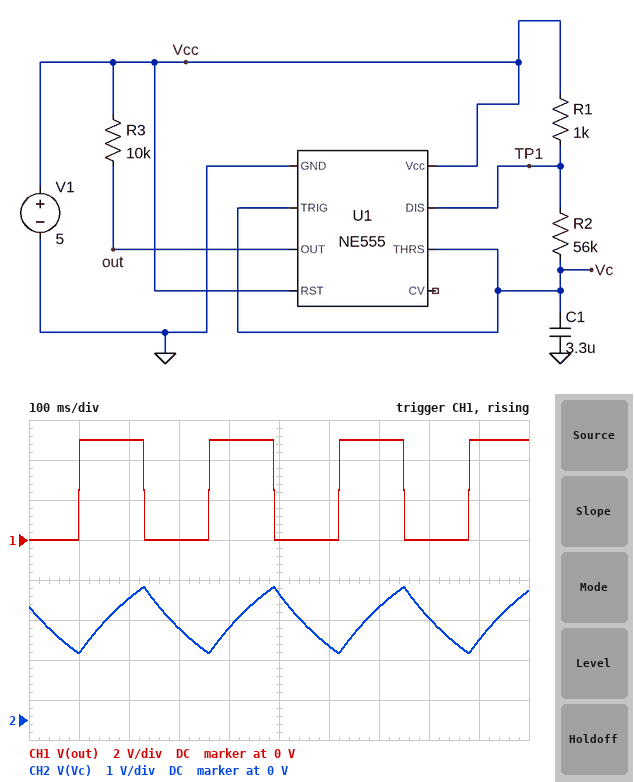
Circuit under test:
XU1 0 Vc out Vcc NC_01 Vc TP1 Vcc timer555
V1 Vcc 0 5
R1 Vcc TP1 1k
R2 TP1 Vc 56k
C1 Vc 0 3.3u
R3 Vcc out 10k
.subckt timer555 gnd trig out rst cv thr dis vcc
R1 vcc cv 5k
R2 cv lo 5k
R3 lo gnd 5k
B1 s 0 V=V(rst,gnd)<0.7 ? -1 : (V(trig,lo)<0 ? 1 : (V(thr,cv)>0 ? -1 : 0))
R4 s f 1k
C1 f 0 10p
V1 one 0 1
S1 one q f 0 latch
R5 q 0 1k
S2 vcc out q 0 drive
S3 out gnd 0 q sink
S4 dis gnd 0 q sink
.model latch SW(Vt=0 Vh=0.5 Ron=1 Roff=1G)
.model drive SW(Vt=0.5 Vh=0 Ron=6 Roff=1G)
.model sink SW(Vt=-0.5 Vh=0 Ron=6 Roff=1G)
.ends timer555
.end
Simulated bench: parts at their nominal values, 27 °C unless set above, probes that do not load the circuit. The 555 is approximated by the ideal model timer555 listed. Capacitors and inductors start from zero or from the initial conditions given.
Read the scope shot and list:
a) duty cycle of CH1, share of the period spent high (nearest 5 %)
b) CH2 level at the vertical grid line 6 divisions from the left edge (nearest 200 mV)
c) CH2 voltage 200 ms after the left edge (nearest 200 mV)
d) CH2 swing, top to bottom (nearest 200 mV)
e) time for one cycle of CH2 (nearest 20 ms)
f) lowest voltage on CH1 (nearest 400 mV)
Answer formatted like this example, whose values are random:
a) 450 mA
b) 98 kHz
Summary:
a) 50 %
b) 1.8 V
c) 3.0 V
d) 1.6 V
e) 260 ms
f) 0 V
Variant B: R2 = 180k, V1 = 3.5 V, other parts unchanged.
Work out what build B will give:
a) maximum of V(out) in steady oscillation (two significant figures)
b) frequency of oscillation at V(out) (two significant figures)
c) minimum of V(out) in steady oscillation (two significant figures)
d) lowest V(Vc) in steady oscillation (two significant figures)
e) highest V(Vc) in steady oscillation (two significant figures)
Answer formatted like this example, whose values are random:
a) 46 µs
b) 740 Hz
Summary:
a) 3.5 V
b) 1.2 Hz
c) 2.1 mV
d) 1.2 V
e) 2.3 V
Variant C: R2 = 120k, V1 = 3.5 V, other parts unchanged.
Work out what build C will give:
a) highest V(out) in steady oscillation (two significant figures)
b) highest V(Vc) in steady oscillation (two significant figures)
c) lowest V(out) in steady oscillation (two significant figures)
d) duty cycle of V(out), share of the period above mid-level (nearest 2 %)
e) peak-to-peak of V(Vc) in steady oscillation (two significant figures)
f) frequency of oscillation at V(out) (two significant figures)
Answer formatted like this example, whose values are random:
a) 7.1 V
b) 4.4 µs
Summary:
a) 3.5 V
b) 2.3 V
c) 2.1 mV
d) 50 %
e) 1.2 V
f) 1.8 Hz
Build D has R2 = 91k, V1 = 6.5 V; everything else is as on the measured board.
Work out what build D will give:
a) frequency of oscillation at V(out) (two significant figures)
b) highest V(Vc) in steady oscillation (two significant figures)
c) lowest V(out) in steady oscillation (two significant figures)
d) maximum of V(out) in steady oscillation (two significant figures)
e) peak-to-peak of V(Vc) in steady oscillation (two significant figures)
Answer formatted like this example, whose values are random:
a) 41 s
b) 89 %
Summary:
a) 2.4 Hz
b) 4.3 V
c) 3.9 mV
d) 6.5 V
e) 2.2 V
